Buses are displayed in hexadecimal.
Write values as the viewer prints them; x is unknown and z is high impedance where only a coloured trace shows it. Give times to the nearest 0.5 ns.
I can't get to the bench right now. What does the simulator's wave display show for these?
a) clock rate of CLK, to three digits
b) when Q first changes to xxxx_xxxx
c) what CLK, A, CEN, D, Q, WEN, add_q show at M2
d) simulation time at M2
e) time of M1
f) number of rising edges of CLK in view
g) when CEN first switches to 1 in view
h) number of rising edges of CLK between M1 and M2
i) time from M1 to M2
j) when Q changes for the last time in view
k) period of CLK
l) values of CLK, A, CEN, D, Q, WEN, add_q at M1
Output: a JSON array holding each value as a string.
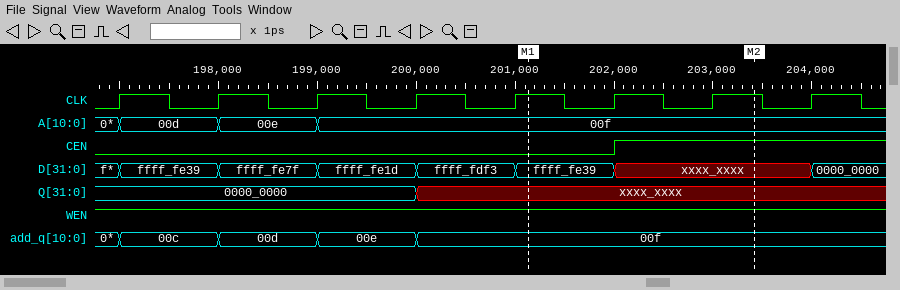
["1.00 GHz", "200 ns", "CLK=1, A=00f, CEN=1, D=xxxx_xxxx, Q=xxxx_xxxx, WEN=1, add_q=00f", "203.5 ns", "201 ns", "8", "202 ns", "2", "2.5 ns", "200 ns", "1 ns", "CLK=1, A=00f, CEN=0, D=ffff_fe39, Q=xxxx_xxxx, WEN=1, add_q=00f"]
